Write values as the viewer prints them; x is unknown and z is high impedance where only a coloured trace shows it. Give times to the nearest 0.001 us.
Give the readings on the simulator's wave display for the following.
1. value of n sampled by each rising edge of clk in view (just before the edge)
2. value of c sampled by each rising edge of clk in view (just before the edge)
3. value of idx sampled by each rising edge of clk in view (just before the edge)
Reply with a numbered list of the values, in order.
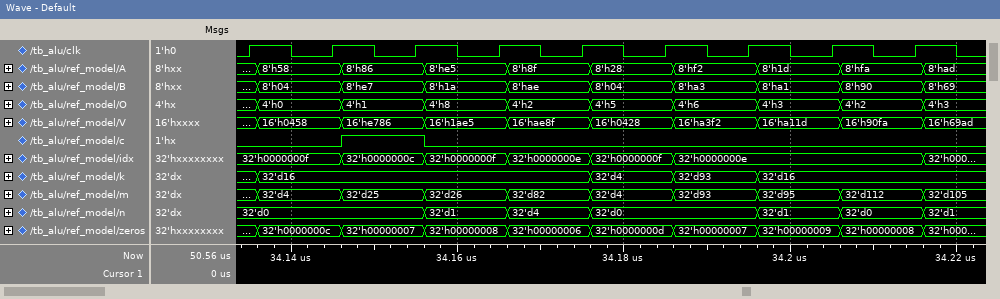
1. 32'd0, 32'd0, 32'd0, 32'd1, 32'd4, 32'd0, 32'd0, 32'd1, 32'd0
2. 0 0 1 0 0 0 0 0 0
3. 32'h0000000f, 32'h0000000f, 32'h0000000c, 32'h0000000f, 32'h0000000e, 32'h0000000f, 32'h0000000e, 32'h0000000e, 32'h0000000e
